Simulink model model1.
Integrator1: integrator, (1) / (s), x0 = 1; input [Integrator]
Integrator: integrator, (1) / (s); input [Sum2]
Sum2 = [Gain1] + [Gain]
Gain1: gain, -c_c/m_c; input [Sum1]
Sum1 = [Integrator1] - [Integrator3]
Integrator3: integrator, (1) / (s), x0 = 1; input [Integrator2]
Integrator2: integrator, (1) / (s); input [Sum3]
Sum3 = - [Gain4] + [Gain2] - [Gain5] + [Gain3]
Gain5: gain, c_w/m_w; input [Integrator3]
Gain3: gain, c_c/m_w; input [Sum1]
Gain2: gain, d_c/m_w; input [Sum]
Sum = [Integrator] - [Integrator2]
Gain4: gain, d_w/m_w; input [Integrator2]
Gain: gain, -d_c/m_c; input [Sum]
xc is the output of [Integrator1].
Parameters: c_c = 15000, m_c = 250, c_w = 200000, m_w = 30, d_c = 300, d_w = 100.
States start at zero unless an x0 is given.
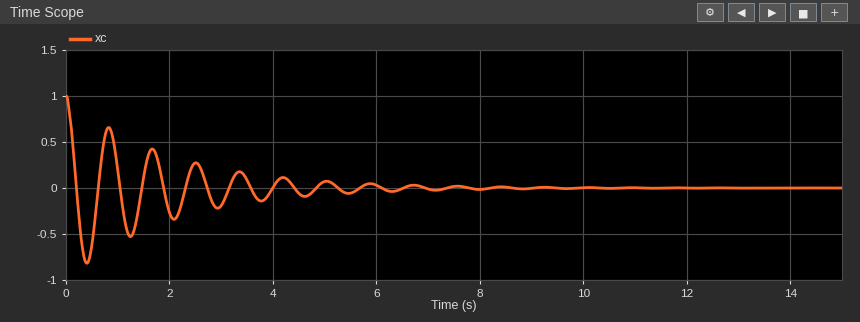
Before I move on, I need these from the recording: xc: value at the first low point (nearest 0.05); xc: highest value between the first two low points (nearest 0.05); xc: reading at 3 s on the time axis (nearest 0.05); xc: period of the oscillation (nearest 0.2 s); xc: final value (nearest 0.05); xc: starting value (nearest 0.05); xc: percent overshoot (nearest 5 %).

-0.80
0.65
-0.20
0.8 s
0.00
1.00
80 %
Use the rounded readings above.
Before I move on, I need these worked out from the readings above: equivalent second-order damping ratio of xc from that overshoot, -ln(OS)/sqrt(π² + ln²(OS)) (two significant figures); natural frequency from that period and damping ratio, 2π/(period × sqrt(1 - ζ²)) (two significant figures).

0.071
7.9 rad/s
